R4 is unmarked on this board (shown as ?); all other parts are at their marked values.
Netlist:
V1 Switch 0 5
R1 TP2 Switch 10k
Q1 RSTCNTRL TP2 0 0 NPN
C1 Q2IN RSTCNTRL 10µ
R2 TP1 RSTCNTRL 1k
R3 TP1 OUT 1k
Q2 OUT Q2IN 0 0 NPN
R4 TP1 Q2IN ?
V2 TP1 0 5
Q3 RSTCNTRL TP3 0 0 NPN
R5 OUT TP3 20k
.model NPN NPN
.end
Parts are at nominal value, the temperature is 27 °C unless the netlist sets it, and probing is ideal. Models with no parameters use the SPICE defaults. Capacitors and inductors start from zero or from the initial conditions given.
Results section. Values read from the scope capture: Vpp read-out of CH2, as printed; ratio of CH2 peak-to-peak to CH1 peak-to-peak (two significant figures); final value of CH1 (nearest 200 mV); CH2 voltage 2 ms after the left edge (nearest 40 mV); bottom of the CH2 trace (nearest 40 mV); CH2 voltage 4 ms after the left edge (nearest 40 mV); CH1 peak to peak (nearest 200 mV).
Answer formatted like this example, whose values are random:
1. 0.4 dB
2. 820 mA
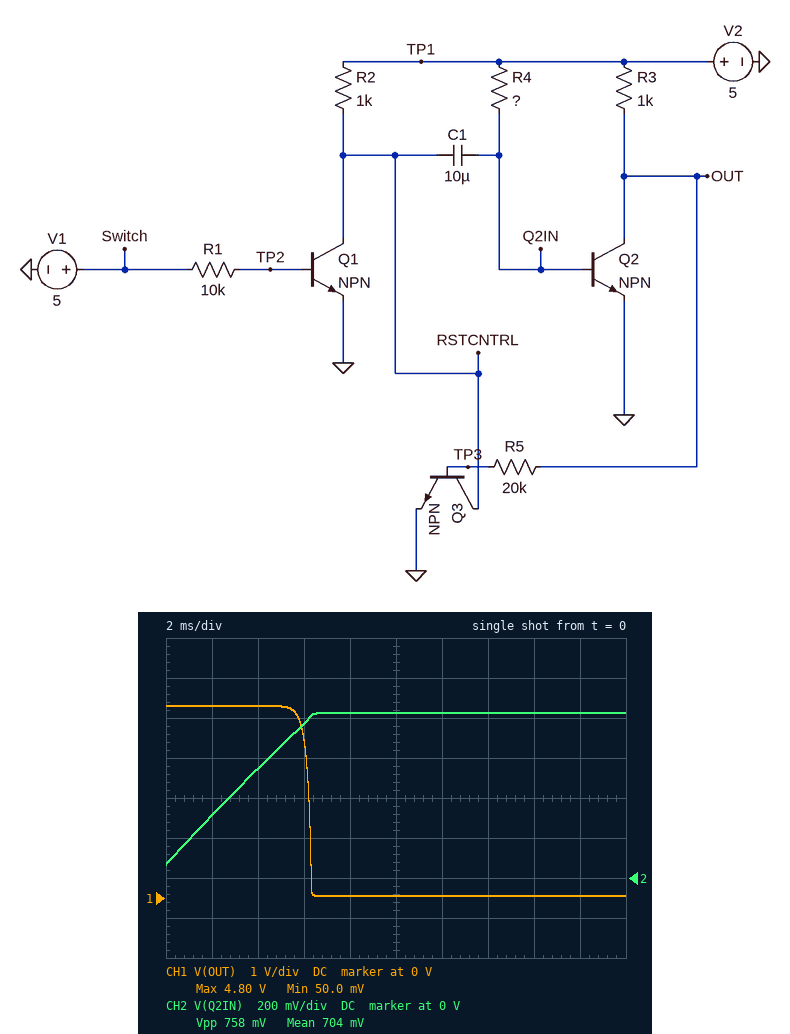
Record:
1. 758 mV
2. 0.16
3. 0 V
4. 320 mV
5. 80 mV
6. 560 mV
7. 4.8 V
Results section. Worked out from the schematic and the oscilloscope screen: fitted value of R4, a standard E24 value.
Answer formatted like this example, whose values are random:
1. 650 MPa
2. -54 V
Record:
1. 3.9 kΩ
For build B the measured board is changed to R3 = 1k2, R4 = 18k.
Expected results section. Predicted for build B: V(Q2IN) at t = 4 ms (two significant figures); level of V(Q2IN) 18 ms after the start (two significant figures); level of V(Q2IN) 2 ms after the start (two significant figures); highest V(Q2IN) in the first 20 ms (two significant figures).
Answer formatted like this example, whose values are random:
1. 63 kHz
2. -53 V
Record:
1. 170 mV
2. 530 mV
3. 120 mV
4. 580 mV
